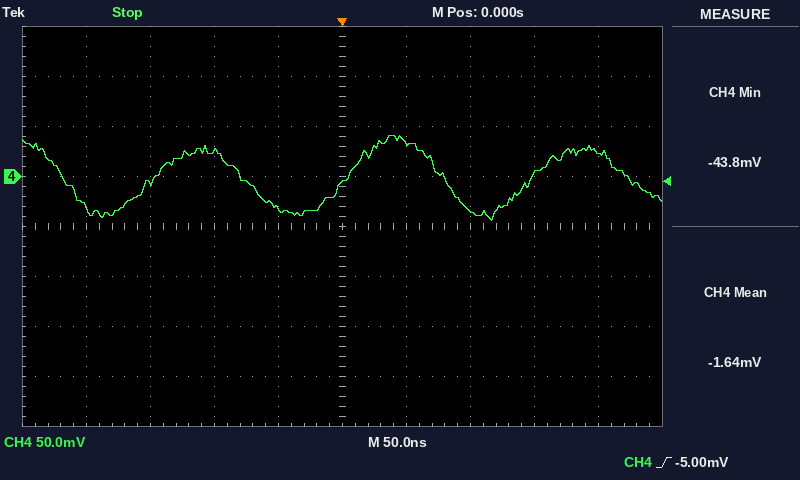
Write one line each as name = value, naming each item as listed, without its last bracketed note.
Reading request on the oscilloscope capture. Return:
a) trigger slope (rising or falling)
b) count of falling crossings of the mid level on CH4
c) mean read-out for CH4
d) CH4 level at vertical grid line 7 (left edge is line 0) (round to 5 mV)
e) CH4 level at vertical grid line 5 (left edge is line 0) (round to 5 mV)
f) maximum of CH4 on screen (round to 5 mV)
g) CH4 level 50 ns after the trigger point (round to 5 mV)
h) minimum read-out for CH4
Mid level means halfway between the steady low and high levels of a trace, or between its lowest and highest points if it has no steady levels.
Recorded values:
trigger slope = rising
count of falling crossings of the mid level on CH4 = 4
mean read-out for CH4 = -1.64 mV
CH4 level at vertical grid line 7 (left edge is line 0) = -35 mV
CH4 level at vertical grid line 5 (left edge is line 0) = -5 mV
maximum of CH4 on screen = 40 mV
CH4 level 50 ns after the trigger point = 35 mV
minimum read-out for CH4 = -43.8 mV
